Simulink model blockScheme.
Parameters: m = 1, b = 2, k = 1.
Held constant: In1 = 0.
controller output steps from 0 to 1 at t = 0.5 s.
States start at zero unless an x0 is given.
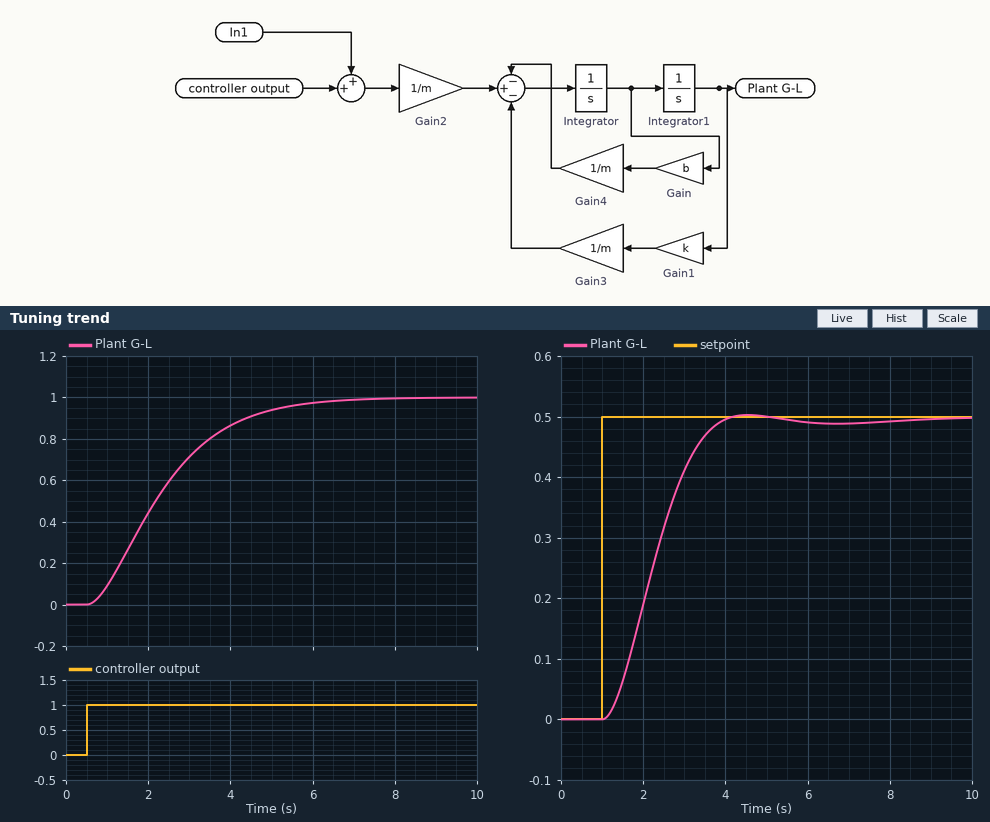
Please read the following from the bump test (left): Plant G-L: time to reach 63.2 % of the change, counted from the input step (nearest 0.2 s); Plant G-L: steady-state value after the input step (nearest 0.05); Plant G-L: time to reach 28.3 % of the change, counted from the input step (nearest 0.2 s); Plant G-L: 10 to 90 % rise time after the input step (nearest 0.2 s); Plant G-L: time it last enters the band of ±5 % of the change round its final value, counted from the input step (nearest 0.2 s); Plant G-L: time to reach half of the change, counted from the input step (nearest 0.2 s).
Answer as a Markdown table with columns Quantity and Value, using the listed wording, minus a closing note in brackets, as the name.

| Quantity | Value |
|---|---|
| Plant G-L: time to reach 63.2 % of the change, counted from the input step | 2.2 s |
| Plant G-L: steady-state value after the input step | 1.00 |
| Plant G-L: time to reach 28.3 % of the change, counted from the input step | 1.0 s |
| Plant G-L: 10 to 90 % rise time after the input step | 3.4 s |
| Plant G-L: time it last enters the band of ±5 % of the change round its final value, counted from the input step | 4.8 s |
| Plant G-L: time to reach half of the change, counted from the input step | 1.6 s |
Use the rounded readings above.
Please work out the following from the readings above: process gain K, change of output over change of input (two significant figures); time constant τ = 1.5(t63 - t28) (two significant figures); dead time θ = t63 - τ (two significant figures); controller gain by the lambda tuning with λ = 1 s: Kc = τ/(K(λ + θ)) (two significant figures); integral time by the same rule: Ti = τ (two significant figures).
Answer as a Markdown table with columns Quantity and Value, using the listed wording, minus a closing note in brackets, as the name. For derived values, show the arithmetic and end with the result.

| Quantity | Value |
|---|---|
| process gain K, change of output over change of input | (1 - 0) / 1 = 1.0 |
| time constant τ = 1.5(t63 - t28) | 1.5 × (2.2 - 1) = 1.8 s |
| dead time θ = t63 - τ | 2.2 - 1.8 = 0.40 s |
| controller gain by the lambda tuning with λ = 1 s: Kc = τ/(K(λ + θ)) | 1.8 / (1 × (1 + 0.4)) = 1.3 |
| integral time by the same rule: Ti = τ | 1.8 s |
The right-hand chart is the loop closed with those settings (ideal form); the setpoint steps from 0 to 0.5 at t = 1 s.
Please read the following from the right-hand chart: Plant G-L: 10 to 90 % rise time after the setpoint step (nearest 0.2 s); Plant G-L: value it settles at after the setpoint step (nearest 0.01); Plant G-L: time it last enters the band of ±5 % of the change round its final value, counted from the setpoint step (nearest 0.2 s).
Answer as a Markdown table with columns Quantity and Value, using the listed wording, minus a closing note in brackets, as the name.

| Quantity | Value |
|---|---|
| Plant G-L: 10 to 90 % rise time after the setpoint step | 1.8 s |
| Plant G-L: value it settles at after the setpoint step | 0.50 |
| Plant G-L: time it last enters the band of ±5 % of the change round its final value, counted from the setpoint step | 2.6 s |
